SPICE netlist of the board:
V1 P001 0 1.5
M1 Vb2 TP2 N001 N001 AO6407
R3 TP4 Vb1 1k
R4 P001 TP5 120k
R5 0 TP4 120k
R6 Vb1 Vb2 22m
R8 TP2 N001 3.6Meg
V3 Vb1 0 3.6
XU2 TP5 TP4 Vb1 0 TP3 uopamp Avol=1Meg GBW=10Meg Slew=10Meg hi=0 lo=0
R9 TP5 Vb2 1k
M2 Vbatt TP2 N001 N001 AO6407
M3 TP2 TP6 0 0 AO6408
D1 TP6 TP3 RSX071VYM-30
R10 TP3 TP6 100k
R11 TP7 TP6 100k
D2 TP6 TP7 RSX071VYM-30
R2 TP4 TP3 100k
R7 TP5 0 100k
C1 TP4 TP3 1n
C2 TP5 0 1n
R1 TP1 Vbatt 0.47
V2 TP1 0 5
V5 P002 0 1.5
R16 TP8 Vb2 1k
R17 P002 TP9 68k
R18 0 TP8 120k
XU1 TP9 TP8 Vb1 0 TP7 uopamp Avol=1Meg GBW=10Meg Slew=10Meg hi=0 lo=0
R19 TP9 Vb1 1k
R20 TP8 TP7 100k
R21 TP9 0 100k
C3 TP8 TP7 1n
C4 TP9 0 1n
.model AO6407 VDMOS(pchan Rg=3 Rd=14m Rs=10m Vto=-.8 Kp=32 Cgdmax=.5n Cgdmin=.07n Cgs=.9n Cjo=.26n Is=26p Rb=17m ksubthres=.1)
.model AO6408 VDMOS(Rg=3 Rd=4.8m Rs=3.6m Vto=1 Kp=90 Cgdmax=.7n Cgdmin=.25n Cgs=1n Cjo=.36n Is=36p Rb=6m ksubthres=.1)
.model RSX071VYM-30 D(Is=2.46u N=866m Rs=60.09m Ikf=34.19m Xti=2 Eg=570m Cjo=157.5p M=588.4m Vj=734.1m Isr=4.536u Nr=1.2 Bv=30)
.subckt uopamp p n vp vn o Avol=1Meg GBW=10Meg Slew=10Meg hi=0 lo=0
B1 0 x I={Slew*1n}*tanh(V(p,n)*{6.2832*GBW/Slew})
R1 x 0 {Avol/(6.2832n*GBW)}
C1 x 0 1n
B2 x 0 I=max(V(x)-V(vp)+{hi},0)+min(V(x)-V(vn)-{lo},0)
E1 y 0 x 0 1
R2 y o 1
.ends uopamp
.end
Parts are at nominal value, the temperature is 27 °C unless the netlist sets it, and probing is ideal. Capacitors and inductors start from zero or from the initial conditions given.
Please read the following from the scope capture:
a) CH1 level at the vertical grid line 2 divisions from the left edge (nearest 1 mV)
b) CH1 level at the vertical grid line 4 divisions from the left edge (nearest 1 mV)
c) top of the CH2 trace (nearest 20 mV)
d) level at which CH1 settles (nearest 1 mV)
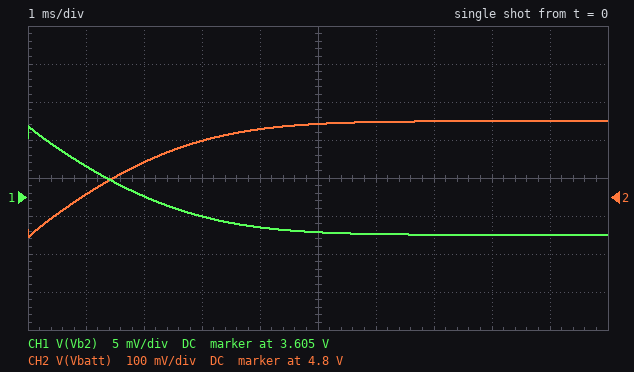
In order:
3.605 V
3.601 V
5.00 V
3.600 V
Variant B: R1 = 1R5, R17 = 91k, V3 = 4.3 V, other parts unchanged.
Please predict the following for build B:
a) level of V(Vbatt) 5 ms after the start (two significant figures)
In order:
4.8 V
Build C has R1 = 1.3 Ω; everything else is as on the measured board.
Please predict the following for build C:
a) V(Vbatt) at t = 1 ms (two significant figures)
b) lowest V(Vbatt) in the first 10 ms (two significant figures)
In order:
4.6 V
4.5 V
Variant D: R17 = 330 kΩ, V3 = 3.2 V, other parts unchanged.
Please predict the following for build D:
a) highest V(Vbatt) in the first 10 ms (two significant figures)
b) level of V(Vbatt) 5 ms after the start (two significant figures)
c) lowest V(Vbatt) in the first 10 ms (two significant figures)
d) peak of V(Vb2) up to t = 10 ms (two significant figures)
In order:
4.7 V
4.6 V
4.5 V
3.2 V
